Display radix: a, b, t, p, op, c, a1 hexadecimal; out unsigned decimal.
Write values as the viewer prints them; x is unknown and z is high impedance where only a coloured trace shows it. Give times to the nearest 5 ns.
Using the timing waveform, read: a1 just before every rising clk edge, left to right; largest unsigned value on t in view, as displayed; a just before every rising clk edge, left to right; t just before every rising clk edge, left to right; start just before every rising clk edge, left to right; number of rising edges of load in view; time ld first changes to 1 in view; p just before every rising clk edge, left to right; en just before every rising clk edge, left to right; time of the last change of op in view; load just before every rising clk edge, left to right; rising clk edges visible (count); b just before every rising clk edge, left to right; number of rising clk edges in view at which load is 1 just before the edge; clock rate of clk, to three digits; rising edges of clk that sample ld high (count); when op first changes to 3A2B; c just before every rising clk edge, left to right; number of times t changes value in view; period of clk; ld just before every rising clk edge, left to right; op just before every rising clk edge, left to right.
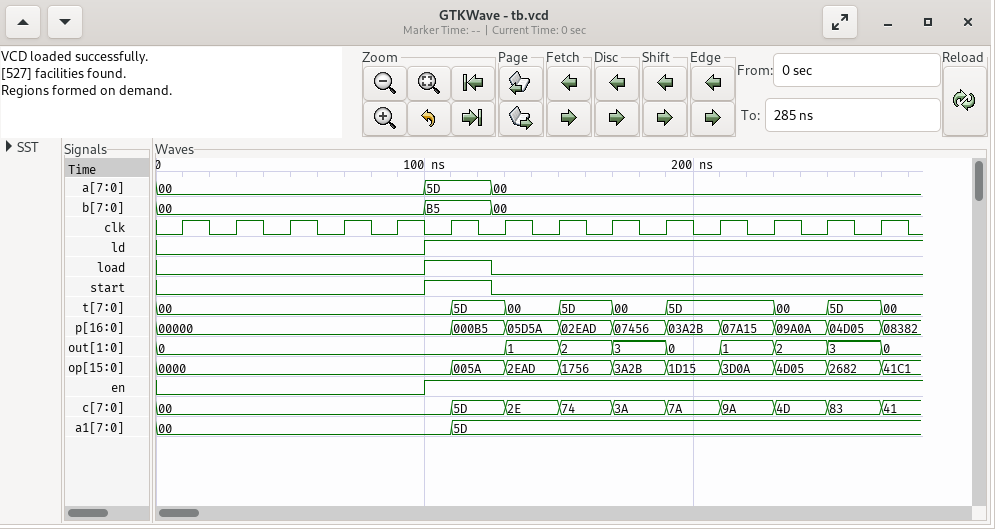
00, 00, 00, 00, 00, 00, 5D, 5D, 5D, 5D, 5D, 5D, 5D, 5D
5D
00, 00, 00, 00, 00, 5D, 00, 00, 00, 00, 00, 00, 00, 00
00, 00, 00, 00, 00, 00, 5D, 00, 5D, 00, 5D, 5D, 00, 5D
0 0 0 0 0 1 0 0 0 0 0 0 0 0
1
100 ns
00000, 00000, 00000, 00000, 00000, 00000, 000B5, 05D5A, 02EAD, 07456, 03A2B, 07A15, 09A0A, 04D05
0 0 0 0 0 1 1 1 1 1 1 1 1 1
270 ns
0 0 0 0 0 1 0 0 0 0 0 0 0 0
14
00, 00, 00, 00, 00, B5, 00, 00, 00, 00, 00, 00, 00, 00
1
50.0 MHz
9
170 ns
00, 00, 00, 00, 00, 00, 5D, 2E, 74, 3A, 7A, 9A, 4D, 83
8
20 ns
0 0 0 0 0 1 1 1 1 1 1 1 1 1
0000, 0000, 0000, 0000, 0000, 0000, 005A, 2EAD, 1756, 3A2B, 1D15, 3D0A, 4D05, 2682
